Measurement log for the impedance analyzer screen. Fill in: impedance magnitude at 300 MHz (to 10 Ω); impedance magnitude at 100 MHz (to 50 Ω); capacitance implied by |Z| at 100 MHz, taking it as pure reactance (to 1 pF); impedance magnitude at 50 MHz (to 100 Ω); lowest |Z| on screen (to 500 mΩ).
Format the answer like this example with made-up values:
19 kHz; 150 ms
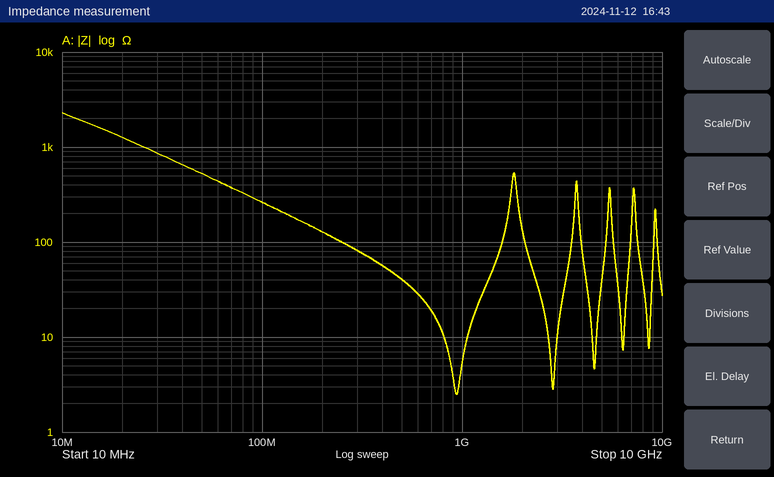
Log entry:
80 Ω; 250 Ω; 6 pF; 500 Ω; 2.5 Ω
